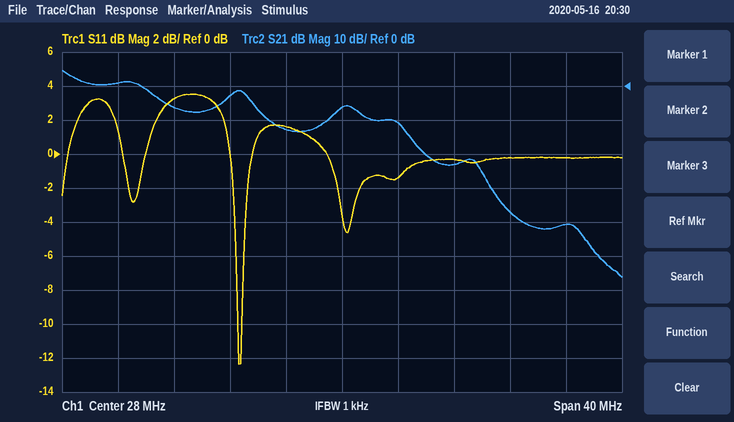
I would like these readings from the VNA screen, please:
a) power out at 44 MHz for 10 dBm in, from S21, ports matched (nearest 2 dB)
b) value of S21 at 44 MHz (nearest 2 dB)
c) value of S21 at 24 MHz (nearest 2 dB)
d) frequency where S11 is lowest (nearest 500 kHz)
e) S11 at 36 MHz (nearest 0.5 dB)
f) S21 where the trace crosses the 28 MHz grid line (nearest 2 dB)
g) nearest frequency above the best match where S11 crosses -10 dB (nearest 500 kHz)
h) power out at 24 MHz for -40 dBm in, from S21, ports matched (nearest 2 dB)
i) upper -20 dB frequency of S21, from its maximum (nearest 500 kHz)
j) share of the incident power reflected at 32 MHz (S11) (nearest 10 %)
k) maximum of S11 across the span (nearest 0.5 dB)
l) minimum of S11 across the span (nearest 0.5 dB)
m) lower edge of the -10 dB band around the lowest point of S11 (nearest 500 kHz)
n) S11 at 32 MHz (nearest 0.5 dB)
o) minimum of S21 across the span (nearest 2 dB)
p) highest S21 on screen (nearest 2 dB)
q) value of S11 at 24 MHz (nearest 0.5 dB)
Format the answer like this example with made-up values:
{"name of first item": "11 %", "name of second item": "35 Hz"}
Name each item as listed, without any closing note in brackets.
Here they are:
{"power out at 44 MHz for 10 dBm in, from S21, ports matched": "-30 dBm", "value of S21 at 44 MHz": "-40 dB", "value of S21 at 24 MHz": "-12 dB", "frequency where S11 is lowest": "20.5 MHz", "S11 at 36 MHz": "-0.5 dB", "S21 where the trace crosses the 28 MHz grid line": "-6 dB", "nearest frequency above the best match where S11 crosses -10 dB": "21.0 MHz", "power out at 24 MHz for -40 dBm in, from S21, ports matched": "-52 dBm", "upper -20 dB frequency of S21, from its maximum": "33.0 MHz", "share of the incident power reflected at 32 MHz (S11)": "70 %", "maximum of S11 across the span": "3.5 dB", "minimum of S11 across the span": "-12.5 dB", "lower edge of the -10 dB band around the lowest point of S11": "20.5 MHz", "S11 at 32 MHz": "-1.5 dB", "minimum of S21 across the span": "-56 dB", "highest S21 on screen": "4 dB", "value of S11 at 24 MHz": "1.5 dB"}
